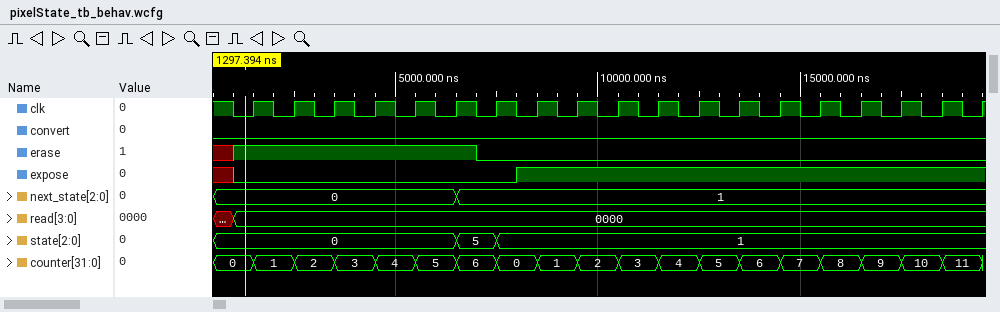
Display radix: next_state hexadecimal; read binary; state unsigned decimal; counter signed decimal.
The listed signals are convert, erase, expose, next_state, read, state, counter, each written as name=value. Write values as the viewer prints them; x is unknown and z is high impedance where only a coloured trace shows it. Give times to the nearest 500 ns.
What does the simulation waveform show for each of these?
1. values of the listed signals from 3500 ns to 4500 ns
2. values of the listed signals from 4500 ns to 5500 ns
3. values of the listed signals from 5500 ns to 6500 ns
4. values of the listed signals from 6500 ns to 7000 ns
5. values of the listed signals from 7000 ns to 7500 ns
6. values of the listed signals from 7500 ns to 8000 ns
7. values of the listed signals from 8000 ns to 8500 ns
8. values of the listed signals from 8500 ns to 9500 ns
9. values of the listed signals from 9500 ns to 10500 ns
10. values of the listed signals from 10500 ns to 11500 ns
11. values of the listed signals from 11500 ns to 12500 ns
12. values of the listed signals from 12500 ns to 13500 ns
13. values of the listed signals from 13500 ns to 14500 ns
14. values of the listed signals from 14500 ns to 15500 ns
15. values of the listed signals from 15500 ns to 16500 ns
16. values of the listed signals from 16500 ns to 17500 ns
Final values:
convert=0, erase=1, expose=0, next_state=0, read=0000, state=0, counter=3
convert=0, erase=1, expose=0, next_state=0, read=0000, state=0, counter=4
convert=0, erase=1, expose=0, next_state=0, read=0000, state=0, counter=5
convert=0, erase=1, expose=0, next_state=1, read=0000, state=5, counter=6
convert=0, erase=0, expose=0, next_state=1, read=0000, state=5, counter=6
convert=0, erase=0, expose=0, next_state=1, read=0000, state=1, counter=0
convert=0, erase=0, expose=1, next_state=1, read=0000, state=1, counter=0
convert=0, erase=0, expose=1, next_state=1, read=0000, state=1, counter=1
convert=0, erase=0, expose=1, next_state=1, read=0000, state=1, counter=2
convert=0, erase=0, expose=1, next_state=1, read=0000, state=1, counter=3
convert=0, erase=0, expose=1, next_state=1, read=0000, state=1, counter=4
convert=0, erase=0, expose=1, next_state=1, read=0000, state=1, counter=5
convert=0, erase=0, expose=1, next_state=1, read=0000, state=1, counter=6
convert=0, erase=0, expose=1, next_state=1, read=0000, state=1, counter=7
convert=0, erase=0, expose=1, next_state=1, read=0000, state=1, counter=8
convert=0, erase=0, expose=1, next_state=1, read=0000, state=1, counter=9
